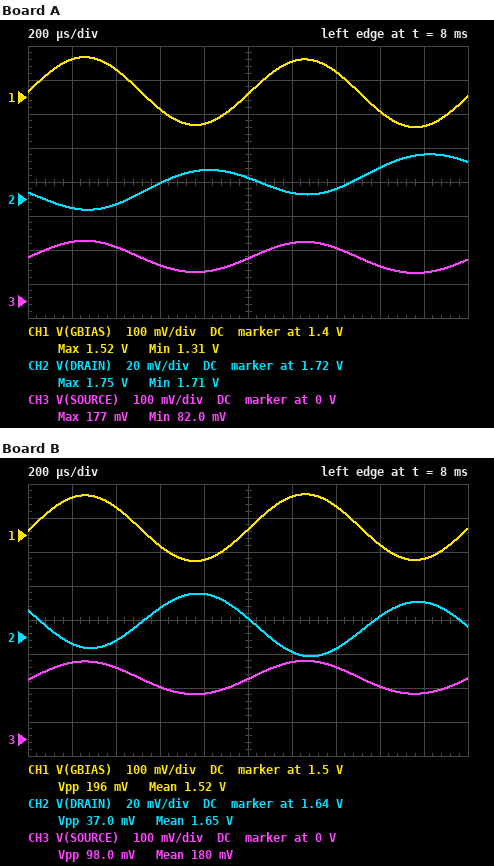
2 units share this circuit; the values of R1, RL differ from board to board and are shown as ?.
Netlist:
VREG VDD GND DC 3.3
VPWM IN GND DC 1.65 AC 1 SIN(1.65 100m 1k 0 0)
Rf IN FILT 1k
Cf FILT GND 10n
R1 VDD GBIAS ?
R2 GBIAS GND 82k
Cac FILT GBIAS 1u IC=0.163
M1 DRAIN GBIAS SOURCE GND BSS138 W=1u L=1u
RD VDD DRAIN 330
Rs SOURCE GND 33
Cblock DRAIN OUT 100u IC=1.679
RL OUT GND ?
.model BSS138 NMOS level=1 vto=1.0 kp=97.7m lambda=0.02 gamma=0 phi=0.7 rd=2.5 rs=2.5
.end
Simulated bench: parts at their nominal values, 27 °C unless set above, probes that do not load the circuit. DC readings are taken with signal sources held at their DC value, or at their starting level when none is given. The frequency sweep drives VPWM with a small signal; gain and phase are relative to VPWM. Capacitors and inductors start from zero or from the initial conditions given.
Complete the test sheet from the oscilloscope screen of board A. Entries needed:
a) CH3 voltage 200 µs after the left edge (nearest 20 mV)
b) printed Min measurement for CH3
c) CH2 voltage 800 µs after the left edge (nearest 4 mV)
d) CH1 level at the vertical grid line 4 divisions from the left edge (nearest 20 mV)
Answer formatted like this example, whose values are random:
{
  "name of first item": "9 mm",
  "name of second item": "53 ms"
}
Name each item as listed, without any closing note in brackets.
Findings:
{
  "CH3 voltage 200 µs after the left edge": "180 mV",
  "printed Min measurement for CH3": "82.0 mV",
  "CH2 voltage 800 µs after the left edge": "1.736 V",
  "CH1 level at the vertical grid line 4 divisions from the left edge": "1.32 V"
}
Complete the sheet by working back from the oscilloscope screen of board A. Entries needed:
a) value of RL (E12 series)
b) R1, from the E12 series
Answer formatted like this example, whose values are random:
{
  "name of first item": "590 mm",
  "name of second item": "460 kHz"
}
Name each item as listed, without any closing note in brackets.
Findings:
{
  "value of RL": "6.8 Ω",
  "R1, from the E12 series": "180 kΩ"
}
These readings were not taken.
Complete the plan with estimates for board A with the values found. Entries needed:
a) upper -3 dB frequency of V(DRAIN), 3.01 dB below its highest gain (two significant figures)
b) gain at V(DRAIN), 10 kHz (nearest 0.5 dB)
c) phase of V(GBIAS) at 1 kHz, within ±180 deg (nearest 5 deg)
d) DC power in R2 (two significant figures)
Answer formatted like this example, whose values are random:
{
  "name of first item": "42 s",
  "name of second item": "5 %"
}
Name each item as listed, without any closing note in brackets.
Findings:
{
  "upper -3 dB frequency of V(DRAIN), 3.01 dB below its highest gain": "9.0 Hz",
  "gain at V(DRAIN), 10 kHz": "-36.0 dB",
  "phase of V(GBIAS) at 1 kHz, within ±180 deg": "-5 deg",
  "DC power in R2": "13 µW"
}
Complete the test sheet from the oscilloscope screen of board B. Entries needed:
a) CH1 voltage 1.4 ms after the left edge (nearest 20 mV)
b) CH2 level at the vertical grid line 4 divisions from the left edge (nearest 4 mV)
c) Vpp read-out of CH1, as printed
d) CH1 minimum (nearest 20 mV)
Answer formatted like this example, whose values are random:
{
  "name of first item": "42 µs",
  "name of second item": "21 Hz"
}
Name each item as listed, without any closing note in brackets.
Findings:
{
  "CH1 voltage 1.4 ms after the left edge": "1.58 V",
  "CH2 level at the vertical grid line 4 divisions from the left edge": "1.664 V",
  "Vpp read-out of CH1, as printed": "196 mV",
  "CH1 minimum": "1.42 V"
}
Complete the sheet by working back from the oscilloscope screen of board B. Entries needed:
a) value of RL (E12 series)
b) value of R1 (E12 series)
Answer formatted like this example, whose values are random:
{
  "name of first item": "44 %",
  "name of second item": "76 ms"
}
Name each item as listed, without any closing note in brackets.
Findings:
{
  "value of RL": "12 Ω",
  "value of R1": "82 kΩ"
}
